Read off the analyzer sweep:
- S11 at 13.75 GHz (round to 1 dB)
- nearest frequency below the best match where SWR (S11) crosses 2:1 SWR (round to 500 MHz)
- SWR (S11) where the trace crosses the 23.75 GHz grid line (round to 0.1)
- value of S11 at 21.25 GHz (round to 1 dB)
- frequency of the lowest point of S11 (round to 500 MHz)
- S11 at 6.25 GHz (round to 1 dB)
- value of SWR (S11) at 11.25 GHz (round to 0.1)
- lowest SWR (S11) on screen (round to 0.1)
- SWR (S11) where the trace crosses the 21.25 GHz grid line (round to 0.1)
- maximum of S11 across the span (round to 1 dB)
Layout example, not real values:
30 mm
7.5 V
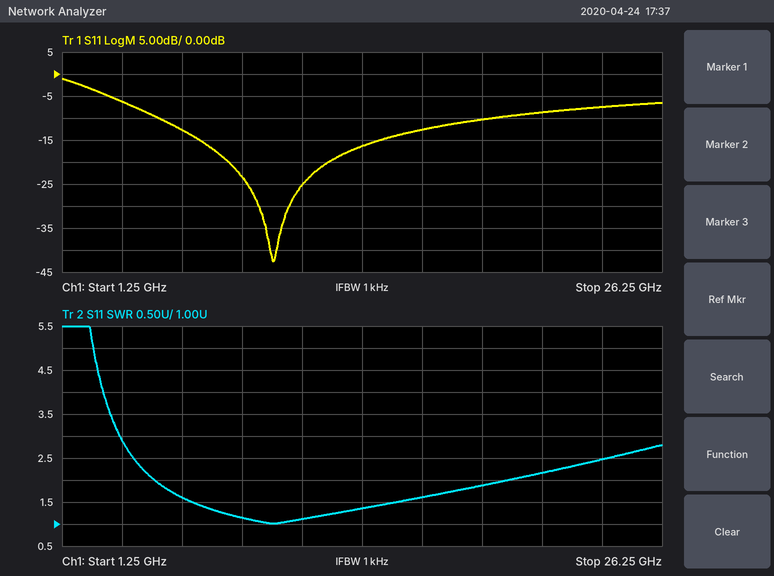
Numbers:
-16 dB
5.0 GHz
2.5
-9 dB
10.0 GHz
-13 dB
1.1
1.0
2.2
-1 dB
